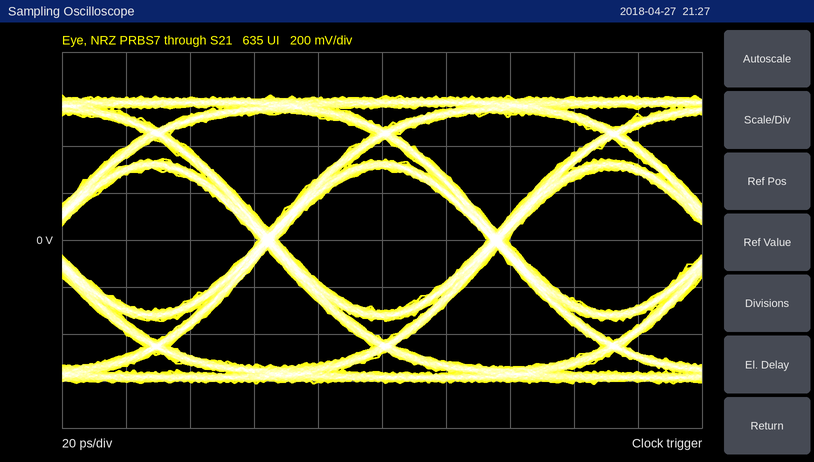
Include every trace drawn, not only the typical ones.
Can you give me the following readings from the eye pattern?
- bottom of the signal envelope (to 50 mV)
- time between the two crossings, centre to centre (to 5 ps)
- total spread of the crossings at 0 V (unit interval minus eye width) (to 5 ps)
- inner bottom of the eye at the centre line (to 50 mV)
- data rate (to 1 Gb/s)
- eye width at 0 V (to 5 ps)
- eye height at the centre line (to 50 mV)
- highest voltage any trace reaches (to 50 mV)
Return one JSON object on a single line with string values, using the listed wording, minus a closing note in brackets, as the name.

{"bottom of the signal envelope": "-600 mV", "time between the two crossings, centre to centre": "70 ps", "total spread of the crossings at 0 V (unit interval minus eye width)": "5 ps", "inner bottom of the eye at the centre line": "-300 mV", "data rate": "14 Gb/s", "eye width at 0 V": "65 ps", "eye height at the centre line": "600 mV", "highest voltage any trace reaches": "600 mV"}
